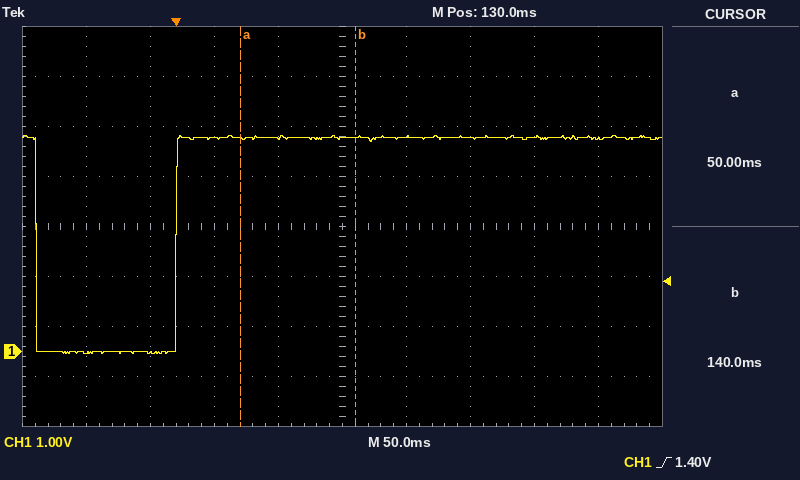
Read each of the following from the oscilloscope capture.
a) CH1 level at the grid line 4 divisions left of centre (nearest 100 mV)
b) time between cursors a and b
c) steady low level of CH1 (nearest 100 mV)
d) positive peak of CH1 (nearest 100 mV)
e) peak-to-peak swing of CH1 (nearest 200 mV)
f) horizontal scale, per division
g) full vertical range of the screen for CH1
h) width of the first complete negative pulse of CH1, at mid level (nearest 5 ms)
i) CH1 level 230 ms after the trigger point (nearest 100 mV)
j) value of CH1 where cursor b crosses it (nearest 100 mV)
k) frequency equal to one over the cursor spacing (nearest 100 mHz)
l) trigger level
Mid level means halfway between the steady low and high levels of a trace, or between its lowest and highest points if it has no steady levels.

0.0 V
90 ms
0.0 V
4.3 V
4.4 V
50 ms
8 V
110 ms
4.3 V
4.3 V
11.1 Hz
1.40 V
